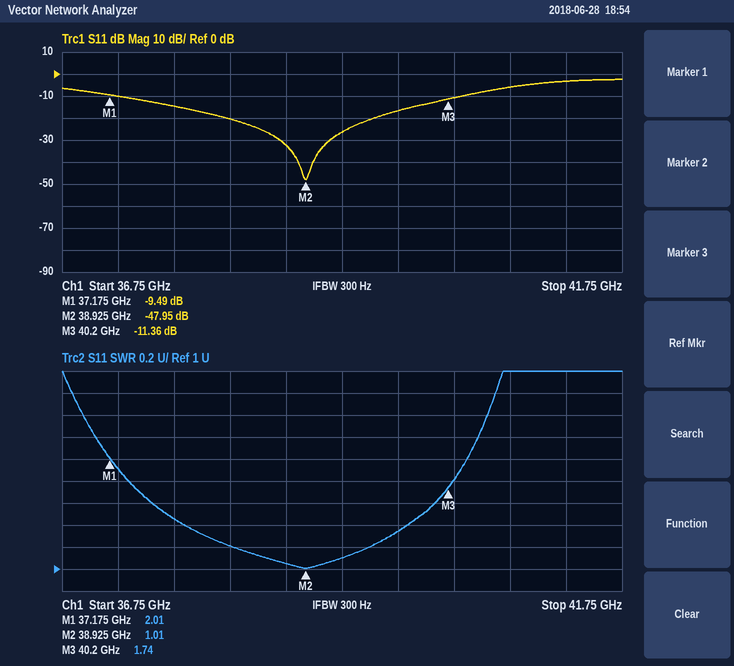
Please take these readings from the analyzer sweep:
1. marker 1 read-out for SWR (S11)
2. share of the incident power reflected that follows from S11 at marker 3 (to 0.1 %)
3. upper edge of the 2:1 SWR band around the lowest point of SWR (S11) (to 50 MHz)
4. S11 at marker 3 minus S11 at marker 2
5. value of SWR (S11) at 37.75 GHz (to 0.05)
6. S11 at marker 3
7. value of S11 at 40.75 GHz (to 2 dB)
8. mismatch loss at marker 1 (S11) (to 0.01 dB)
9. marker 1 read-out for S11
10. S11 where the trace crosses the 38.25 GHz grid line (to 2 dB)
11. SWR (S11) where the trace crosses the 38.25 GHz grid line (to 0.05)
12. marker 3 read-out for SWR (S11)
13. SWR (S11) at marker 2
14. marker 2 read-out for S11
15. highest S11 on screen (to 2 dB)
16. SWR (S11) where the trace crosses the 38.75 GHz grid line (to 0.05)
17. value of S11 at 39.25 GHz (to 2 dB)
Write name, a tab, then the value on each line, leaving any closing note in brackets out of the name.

marker 1 read-out for SWR	2.01
share of the incident power reflected that follows from S11 at marker 3	7.3 %
upper edge of the 2:1 SWR band around the lowest point of SWR (S11)	40.35 GHz
S11 at marker 3 minus S11 at marker 2	36.59 dB
value of SWR (S11) at 37.75 GHz	1.45
S11 at marker 3	-11.36 dB
value of S11 at 40.75 GHz	-6 dB
mismatch loss at marker 1 (S11)	0.52 dB
marker 1 read-out for S11	-9.49 dB
S11 where the trace crosses the 38.25 GHz grid line	-20 dB
SWR (S11) where the trace crosses the 38.25 GHz grid line	1.20
marker 3 read-out for SWR	1.74
SWR (S11) at marker 2	1.01
marker 2 read-out for S11	-47.95 dB
highest S11 on screen	-2 dB
SWR (S11) where the trace crosses the 38.75 GHz grid line	1.05
value of S11 at 39.25 GHz	-26 dB
